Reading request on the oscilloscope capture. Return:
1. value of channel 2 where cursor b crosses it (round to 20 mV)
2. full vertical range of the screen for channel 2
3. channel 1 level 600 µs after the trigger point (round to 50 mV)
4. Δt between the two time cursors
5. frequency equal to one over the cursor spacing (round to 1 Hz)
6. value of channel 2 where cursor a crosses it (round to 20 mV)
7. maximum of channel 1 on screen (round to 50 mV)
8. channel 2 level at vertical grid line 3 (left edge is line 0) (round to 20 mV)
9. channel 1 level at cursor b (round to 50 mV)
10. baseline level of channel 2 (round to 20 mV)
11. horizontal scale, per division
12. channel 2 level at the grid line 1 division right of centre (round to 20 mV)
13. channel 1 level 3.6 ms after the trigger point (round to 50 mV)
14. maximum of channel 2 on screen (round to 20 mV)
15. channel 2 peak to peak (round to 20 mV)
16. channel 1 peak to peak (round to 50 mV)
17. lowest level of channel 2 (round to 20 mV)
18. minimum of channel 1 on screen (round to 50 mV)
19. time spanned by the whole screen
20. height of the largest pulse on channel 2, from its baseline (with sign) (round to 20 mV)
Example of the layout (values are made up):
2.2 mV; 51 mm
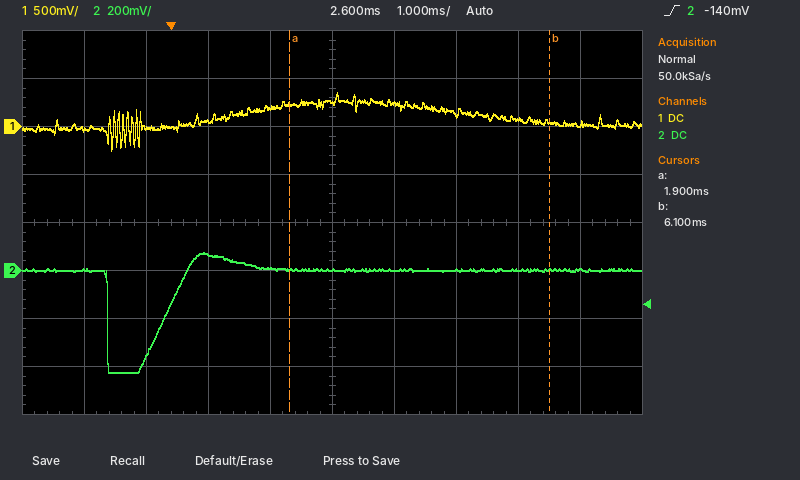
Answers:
0 mV; 1.6 V; 50 mV; 4.2 ms; 238 Hz; 0 mV; 350 mV; 60 mV; 50 mV; 0 mV; 1 ms; 0 mV; 250 mV; 80 mV; 500 mV; 600 mV; -420 mV; -250 mV; 10 ms; -420 mV
